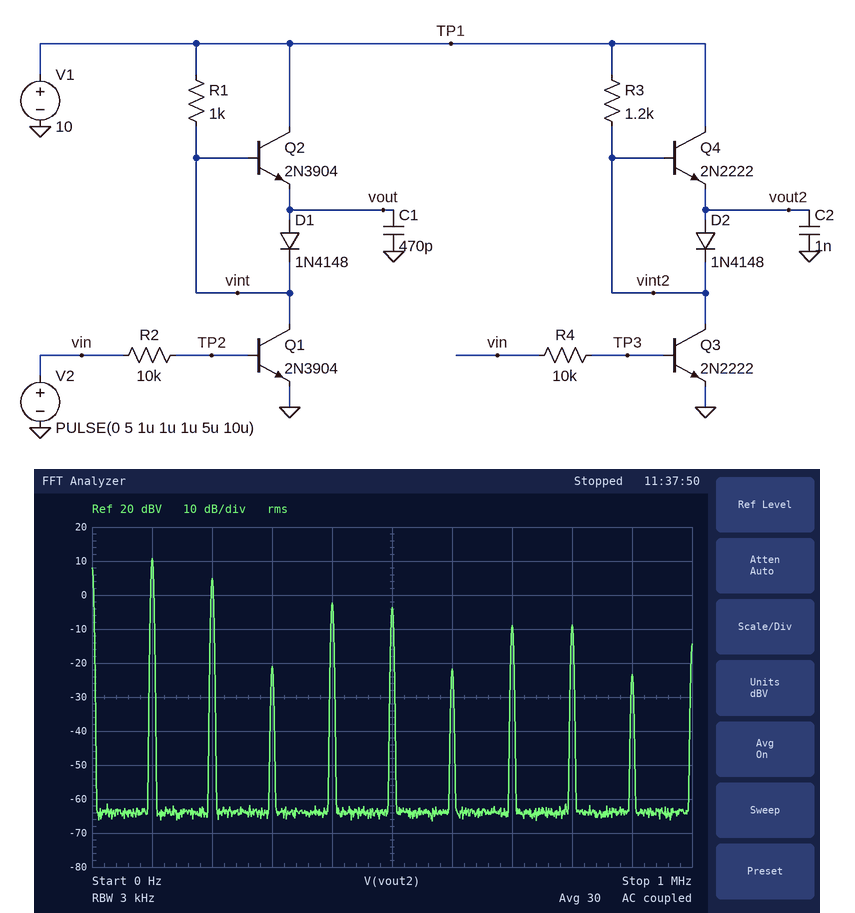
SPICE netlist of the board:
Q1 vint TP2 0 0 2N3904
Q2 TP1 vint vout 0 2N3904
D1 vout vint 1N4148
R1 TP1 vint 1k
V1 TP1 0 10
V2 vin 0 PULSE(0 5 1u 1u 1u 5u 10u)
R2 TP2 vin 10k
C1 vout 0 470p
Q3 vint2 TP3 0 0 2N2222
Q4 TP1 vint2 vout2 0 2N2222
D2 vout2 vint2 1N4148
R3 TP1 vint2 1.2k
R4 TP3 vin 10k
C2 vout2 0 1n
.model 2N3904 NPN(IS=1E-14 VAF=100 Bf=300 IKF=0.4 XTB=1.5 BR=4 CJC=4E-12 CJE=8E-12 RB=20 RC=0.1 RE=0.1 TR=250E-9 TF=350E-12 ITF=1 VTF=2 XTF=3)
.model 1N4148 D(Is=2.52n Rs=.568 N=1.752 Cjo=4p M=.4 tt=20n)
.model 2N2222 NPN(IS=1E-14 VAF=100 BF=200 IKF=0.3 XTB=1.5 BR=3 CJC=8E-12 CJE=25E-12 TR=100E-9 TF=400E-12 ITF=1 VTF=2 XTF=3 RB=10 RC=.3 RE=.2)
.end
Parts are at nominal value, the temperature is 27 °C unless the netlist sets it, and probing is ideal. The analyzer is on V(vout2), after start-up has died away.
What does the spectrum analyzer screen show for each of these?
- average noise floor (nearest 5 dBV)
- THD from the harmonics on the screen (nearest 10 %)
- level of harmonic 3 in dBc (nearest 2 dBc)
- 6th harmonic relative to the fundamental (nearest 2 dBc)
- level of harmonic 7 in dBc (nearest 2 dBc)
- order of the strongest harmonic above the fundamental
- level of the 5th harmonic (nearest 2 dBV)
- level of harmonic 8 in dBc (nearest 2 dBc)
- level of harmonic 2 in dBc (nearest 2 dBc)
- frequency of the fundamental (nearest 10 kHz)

-65 dBV
60 %
-32 dBc
-32 dBc
-20 dBc
2
-4 dBV
-20 dBc
-6 dBc
100 kHz
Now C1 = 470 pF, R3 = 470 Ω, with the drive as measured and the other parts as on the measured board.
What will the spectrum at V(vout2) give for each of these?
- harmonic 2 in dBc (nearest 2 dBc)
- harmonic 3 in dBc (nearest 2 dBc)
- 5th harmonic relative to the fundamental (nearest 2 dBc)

-8 dBc
-24 dBc
-18 dBc
